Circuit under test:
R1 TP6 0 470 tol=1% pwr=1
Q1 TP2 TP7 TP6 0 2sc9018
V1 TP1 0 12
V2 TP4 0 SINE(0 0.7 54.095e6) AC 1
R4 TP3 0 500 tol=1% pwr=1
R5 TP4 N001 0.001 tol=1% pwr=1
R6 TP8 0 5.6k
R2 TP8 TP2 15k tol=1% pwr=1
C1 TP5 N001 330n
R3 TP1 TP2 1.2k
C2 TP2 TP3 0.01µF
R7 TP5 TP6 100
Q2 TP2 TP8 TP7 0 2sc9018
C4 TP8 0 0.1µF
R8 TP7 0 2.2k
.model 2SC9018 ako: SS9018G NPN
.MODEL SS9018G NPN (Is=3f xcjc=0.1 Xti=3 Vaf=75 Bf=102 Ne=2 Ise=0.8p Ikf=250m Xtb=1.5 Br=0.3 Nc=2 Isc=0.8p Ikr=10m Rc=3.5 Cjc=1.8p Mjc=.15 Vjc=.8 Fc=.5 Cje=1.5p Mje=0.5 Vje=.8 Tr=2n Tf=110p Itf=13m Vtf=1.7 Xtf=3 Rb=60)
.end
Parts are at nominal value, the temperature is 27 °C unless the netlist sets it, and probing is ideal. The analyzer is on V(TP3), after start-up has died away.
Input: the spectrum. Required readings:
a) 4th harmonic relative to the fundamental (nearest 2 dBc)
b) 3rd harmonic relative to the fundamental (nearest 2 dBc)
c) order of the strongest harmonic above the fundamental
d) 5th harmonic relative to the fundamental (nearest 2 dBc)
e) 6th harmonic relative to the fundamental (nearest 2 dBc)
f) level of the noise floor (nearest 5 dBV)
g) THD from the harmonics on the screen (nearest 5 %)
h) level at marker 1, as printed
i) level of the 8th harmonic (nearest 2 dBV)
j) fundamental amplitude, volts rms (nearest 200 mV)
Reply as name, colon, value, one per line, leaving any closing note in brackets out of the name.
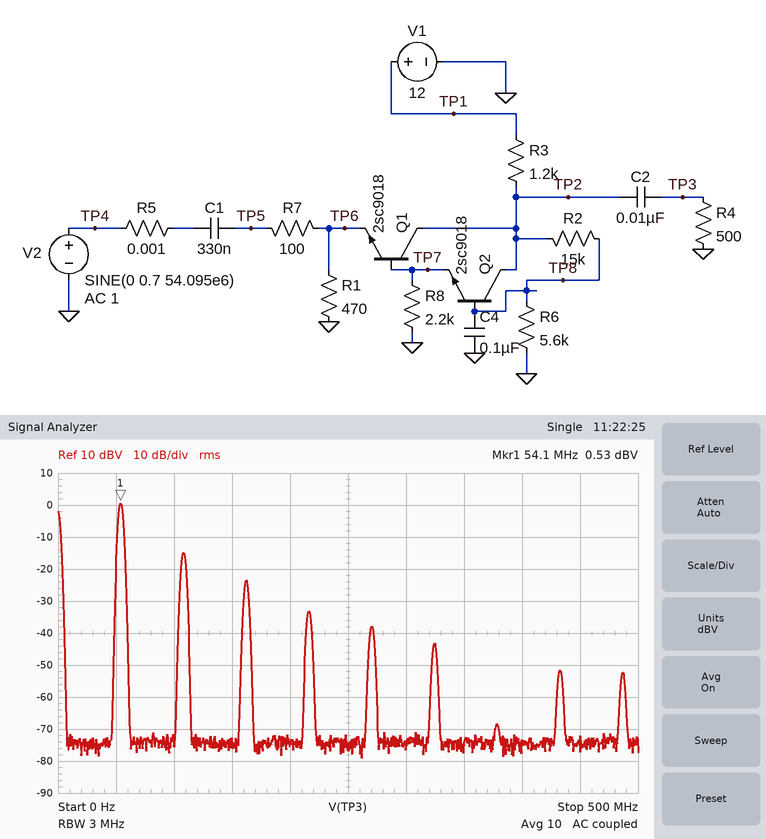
4th harmonic relative to the fundamental: -34 dBc
3rd harmonic relative to the fundamental: -24 dBc
order of the strongest harmonic above the fundamental: 2
5th harmonic relative to the fundamental: -38 dBc
6th harmonic relative to the fundamental: -44 dBc
level of the noise floor: -75 dBV
THD from the harmonics on the screen: 20 %
level at marker 1, as printed: 0.53 dBV
level of the 8th harmonic: -52 dBV
fundamental amplitude, volts rms: 1.0 V
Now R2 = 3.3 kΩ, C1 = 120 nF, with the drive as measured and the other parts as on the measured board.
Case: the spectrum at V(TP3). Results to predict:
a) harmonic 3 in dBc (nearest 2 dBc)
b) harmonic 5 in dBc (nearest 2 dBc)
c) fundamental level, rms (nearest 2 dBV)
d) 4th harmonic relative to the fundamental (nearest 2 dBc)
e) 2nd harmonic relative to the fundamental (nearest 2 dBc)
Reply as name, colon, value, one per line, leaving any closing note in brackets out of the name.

harmonic 3 in dBc: -26 dBc
harmonic 5 in dBc: -40 dBc
fundamental level, rms: 2 dBV
4th harmonic relative to the fundamental: -32 dBc
2nd harmonic relative to the fundamental: -22 dBc
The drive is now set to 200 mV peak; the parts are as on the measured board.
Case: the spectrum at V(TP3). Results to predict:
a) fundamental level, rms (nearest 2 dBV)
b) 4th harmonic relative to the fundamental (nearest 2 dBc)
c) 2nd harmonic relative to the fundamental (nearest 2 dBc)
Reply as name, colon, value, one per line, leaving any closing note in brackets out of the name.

fundamental level, rms: -8 dBV
4th harmonic relative to the fundamental: -52 dBc
2nd harmonic relative to the fundamental: -30 dBc
